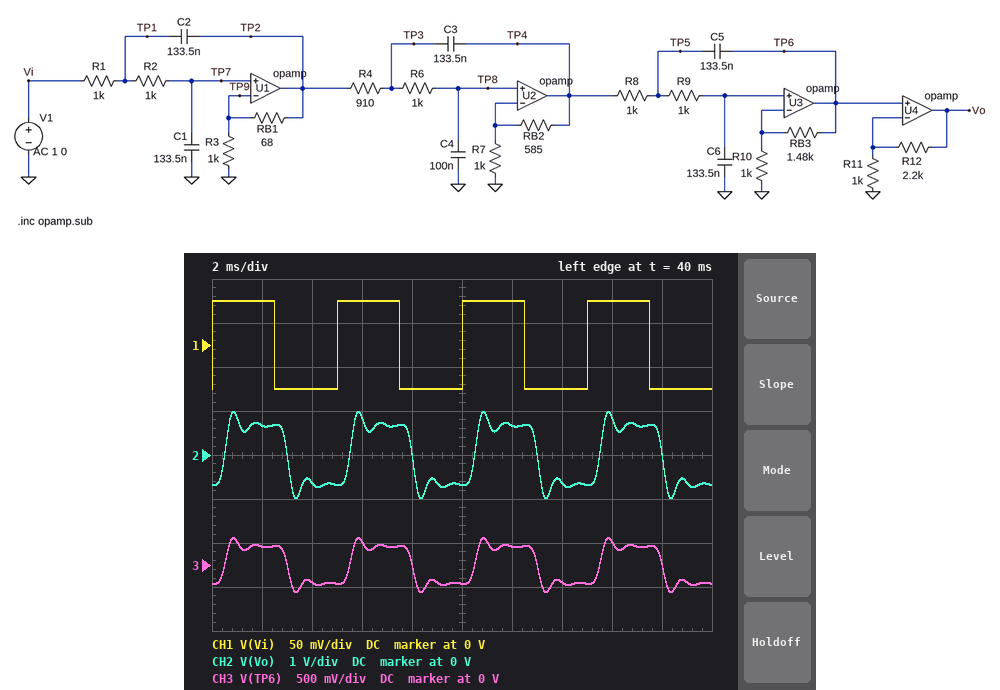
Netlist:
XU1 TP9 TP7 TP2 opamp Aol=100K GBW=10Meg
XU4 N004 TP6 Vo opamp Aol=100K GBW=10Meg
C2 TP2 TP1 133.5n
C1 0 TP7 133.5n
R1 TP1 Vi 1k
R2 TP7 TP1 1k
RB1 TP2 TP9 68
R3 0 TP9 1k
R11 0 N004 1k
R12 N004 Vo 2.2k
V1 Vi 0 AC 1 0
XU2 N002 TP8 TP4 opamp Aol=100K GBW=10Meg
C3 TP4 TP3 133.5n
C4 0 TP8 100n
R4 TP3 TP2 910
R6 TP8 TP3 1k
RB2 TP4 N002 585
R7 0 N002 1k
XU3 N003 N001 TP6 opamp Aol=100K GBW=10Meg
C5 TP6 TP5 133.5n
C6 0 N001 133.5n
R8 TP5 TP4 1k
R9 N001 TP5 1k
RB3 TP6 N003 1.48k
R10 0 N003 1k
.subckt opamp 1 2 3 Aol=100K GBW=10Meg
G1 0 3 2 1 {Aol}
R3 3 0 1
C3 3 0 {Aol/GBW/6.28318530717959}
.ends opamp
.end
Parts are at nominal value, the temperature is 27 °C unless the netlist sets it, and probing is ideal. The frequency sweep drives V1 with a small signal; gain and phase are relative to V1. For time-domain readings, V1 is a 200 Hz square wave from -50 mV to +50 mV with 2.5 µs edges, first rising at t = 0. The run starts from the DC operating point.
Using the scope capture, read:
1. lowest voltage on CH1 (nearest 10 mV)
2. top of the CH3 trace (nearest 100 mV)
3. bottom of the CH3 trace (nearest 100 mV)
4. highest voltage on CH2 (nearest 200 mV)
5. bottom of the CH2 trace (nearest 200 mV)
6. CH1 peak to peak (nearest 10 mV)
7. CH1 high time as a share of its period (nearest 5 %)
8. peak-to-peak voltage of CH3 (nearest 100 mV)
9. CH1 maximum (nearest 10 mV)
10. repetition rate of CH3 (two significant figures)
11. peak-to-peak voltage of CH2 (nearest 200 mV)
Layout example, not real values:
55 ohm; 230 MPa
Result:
-50 mV; 300 mV; -300 mV; 1.0 V; -1.0 V; 100 mV; 50 %; 600 mV; 50 mV; 200 Hz; 2.0 V
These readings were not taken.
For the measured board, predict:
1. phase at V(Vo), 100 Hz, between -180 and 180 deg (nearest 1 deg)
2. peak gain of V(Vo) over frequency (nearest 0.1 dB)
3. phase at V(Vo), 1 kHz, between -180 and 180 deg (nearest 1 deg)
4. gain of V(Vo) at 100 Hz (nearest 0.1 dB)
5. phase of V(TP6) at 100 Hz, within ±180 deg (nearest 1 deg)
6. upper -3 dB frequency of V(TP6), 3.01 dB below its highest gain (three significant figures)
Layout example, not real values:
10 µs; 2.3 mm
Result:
-16 deg; 24.6 dB; 169 deg; 22.6 dB; -16 deg; 1.26 kHz
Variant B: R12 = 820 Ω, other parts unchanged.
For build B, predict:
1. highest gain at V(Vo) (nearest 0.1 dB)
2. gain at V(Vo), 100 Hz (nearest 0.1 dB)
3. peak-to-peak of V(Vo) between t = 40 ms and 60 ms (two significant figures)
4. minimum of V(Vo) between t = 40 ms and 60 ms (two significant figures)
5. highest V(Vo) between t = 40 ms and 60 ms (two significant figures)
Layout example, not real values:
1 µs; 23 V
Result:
19.7 dB; 17.7 dB; 1.1 V; -560 mV; 560 mV
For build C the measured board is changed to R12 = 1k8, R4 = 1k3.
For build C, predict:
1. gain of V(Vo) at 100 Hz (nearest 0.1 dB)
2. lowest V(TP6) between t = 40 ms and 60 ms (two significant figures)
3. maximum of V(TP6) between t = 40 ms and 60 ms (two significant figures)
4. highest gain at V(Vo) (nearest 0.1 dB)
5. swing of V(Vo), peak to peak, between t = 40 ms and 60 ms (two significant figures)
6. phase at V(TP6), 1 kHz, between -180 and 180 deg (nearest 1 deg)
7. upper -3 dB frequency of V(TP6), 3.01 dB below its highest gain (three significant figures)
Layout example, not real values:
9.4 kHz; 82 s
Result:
21.4 dB; -320 mV; 320 mV; 23.9 dB; 1.8 V; 156 deg; 1.23 kHz
